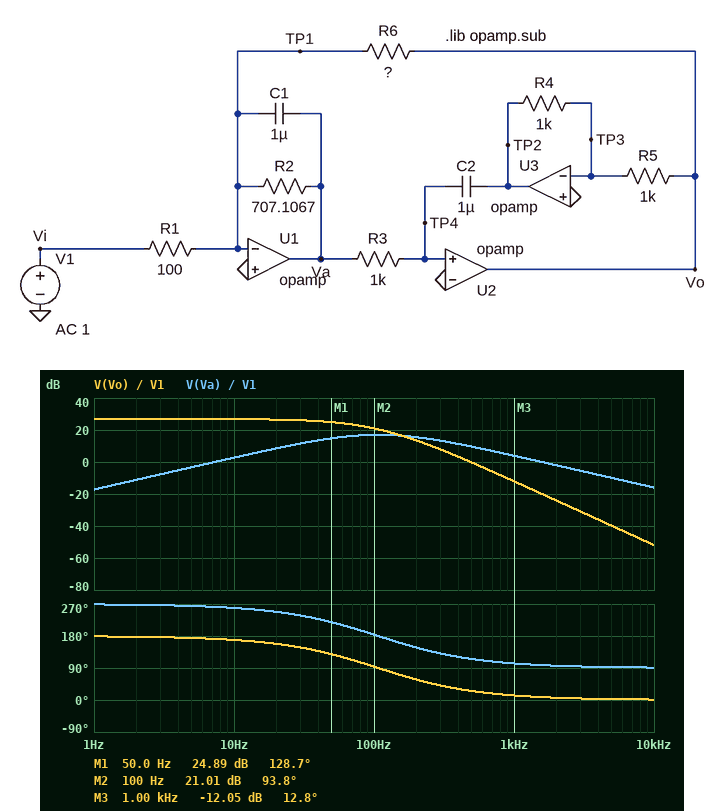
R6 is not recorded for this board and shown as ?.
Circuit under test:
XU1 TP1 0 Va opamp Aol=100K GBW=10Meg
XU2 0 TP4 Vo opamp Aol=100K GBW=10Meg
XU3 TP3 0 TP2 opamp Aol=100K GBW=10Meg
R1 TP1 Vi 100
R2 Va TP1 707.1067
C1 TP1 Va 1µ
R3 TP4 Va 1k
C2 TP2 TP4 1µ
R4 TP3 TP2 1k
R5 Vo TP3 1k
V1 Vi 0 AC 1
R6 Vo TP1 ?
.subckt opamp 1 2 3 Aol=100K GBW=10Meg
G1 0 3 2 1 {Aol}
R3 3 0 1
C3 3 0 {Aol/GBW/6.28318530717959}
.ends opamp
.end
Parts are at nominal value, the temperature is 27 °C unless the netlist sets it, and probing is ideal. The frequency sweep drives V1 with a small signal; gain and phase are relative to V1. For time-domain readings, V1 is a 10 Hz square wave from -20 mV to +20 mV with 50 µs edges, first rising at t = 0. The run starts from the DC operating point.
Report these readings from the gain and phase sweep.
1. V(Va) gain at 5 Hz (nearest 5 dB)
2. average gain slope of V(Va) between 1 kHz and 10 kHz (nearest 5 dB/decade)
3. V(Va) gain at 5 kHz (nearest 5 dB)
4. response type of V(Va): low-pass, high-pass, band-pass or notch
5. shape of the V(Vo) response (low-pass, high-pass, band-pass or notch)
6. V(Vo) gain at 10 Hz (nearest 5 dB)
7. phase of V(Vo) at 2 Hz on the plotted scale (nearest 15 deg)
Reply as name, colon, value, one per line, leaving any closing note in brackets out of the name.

V(Va) gain at 5 Hz: -5 dB
average gain slope of V(Va) between 1 kHz and 10 kHz: -20 dB/decade
V(Va) gain at 5 kHz: -10 dB
response type of V(Va): low-pass, high-pass, band-pass or notch: band-pass
shape of the V(Vo) response: low-pass
V(Vo) gain at 10 Hz: 25 dB
phase of V(Vo) at 2 Hz on the plotted scale: 180 deg
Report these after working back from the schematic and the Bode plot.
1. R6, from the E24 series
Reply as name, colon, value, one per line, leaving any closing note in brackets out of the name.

R6, from the E24 series: 2.2 kΩ
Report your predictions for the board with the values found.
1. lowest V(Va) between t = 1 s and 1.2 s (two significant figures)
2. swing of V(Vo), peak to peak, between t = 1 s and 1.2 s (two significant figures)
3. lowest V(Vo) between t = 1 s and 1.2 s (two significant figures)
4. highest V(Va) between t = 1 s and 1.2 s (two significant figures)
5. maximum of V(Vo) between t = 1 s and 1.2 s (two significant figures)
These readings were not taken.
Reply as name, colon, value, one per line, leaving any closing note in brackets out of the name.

lowest V(Va) between t = 1 s and 1.2 s: -210 mV
swing of V(Vo), peak to peak, between t = 1 s and 1.2 s: 880 mV
lowest V(Vo) between t = 1 s and 1.2 s: -440 mV
highest V(Va) between t = 1 s and 1.2 s: 210 mV
maximum of V(Vo) between t = 1 s and 1.2 s: 440 mV
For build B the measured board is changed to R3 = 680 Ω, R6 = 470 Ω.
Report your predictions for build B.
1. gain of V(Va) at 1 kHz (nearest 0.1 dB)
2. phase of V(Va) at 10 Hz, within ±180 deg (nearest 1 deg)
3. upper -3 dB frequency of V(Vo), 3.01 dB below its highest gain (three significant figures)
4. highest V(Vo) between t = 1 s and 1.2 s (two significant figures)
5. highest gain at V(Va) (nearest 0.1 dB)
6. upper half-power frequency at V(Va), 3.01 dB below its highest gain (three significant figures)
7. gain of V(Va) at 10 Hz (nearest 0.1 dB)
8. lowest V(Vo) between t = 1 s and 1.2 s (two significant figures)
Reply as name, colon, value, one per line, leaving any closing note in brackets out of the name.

gain of V(Va) at 1 kHz: 4.5 dB
phase of V(Va) at 10 Hz, within ±180 deg: -92 deg
upper -3 dB frequency of V(Vo), 3.01 dB below its highest gain: 335 Hz
highest V(Vo) between t = 1 s and 1.2 s: 140 mV
highest gain at V(Va): 17.0 dB
upper half-power frequency at V(Va), 3.01 dB below its highest gain: 416 Hz
gain of V(Va) at 10 Hz: -13.9 dB
lowest V(Vo) between t = 1 s and 1.2 s: -140 mV
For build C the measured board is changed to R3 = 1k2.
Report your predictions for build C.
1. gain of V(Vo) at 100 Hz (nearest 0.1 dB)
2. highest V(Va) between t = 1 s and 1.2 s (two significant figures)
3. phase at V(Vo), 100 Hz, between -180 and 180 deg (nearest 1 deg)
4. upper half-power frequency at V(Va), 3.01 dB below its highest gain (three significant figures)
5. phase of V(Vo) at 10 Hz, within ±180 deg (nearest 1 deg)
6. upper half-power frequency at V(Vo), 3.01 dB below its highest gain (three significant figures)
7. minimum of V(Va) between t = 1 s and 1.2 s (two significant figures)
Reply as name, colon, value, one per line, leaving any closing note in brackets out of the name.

gain of V(Vo) at 100 Hz: 19.4 dB
highest V(Va) between t = 1 s and 1.2 s: 220 mV
phase at V(Vo), 100 Hz, between -180 and 180 deg: 89 deg
upper half-power frequency at V(Va), 3.01 dB below its highest gain: 262 Hz
phase of V(Vo) at 10 Hz, within ±180 deg: 167 deg
upper half-power frequency at V(Vo), 3.01 dB below its highest gain: 51.9 Hz
minimum of V(Va) between t = 1 s and 1.2 s: -220 mV
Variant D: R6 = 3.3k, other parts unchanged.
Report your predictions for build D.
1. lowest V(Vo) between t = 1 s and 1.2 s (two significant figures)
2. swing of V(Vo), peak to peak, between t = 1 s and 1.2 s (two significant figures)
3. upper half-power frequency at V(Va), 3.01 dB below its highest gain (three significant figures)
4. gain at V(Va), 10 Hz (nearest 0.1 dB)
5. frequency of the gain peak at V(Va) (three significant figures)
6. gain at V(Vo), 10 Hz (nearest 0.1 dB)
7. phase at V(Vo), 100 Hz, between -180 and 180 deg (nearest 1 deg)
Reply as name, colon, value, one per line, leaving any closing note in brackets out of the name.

lowest V(Vo) between t = 1 s and 1.2 s: -660 mV
swing of V(Vo), peak to peak, between t = 1 s and 1.2 s: 1.3 V
upper half-power frequency at V(Va), 3.01 dB below its highest gain: 255 Hz
gain at V(Va), 10 Hz: 6.1 dB
frequency of the gain peak at V(Va): 87.6 Hz
gain at V(Vo), 10 Hz: 30.1 dB
phase at V(Vo), 100 Hz, between -180 and 180 deg: 84 deg
